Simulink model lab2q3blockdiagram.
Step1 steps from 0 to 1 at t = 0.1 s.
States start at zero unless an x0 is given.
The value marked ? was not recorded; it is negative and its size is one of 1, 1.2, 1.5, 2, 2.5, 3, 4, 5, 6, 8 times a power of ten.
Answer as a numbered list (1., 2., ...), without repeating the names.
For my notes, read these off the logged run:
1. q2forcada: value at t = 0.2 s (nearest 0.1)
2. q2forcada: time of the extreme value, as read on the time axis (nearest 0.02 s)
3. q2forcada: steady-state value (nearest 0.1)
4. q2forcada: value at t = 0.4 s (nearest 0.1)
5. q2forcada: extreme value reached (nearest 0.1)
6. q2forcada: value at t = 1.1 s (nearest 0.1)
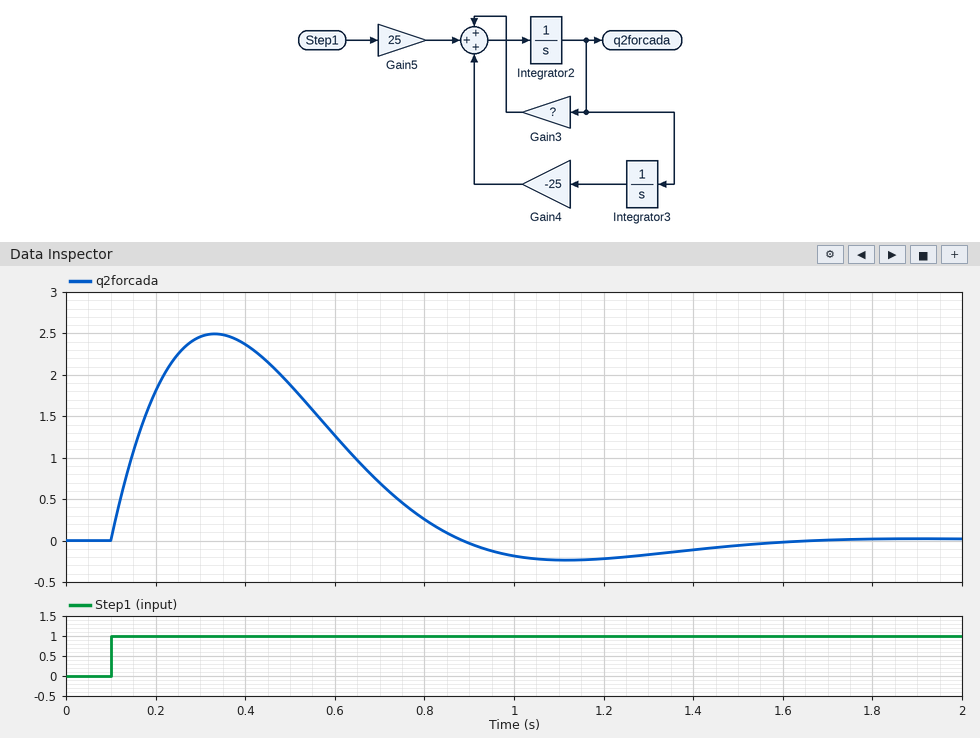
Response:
1. 1.8
2. 0.34 s
3. 0.0
4. 2.4
5. 2.5
6. -0.2
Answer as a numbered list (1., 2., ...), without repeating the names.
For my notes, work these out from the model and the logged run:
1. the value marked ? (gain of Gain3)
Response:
1. -6
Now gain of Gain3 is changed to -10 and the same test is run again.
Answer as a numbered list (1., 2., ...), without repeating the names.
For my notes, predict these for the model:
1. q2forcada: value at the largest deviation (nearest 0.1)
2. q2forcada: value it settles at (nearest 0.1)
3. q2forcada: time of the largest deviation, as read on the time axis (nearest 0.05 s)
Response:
1. 1.8
2. 0.0
3. 0.30 s
